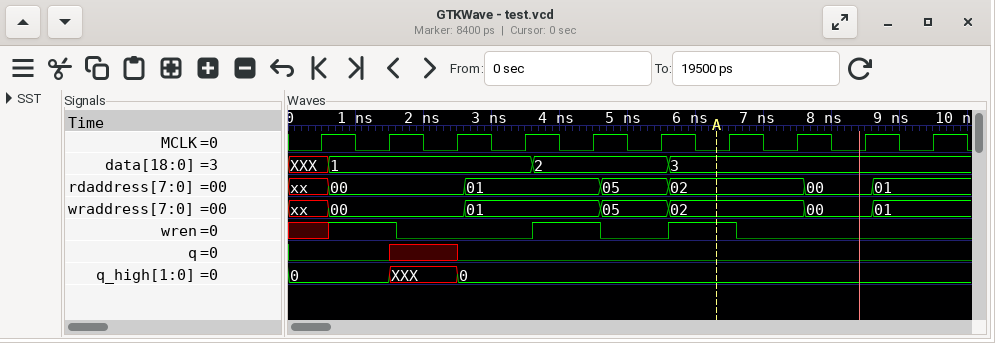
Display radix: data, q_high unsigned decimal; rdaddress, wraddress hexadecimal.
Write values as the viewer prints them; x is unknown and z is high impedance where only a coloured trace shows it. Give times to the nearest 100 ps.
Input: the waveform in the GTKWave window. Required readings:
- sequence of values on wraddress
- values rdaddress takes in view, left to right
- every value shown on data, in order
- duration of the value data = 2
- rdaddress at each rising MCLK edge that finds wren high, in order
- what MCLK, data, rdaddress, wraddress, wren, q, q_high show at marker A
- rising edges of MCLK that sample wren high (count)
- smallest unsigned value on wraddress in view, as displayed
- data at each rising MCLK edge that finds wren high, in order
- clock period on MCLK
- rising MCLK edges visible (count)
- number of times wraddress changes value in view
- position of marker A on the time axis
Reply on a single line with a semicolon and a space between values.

xx, 00, 01, 05, 02, 00, 01; xx, 00, 01, 05, 02, 00, 01; XXX, 1, 2, 3; 2000 ps; 00, 01, 02; MCLK=0, data=3, rdaddress=02, wraddress=02, wren=1, q=0, q_high=0; 3; 00; 1, 2, 3; 1000 ps; 10; 6; 6300 ps
